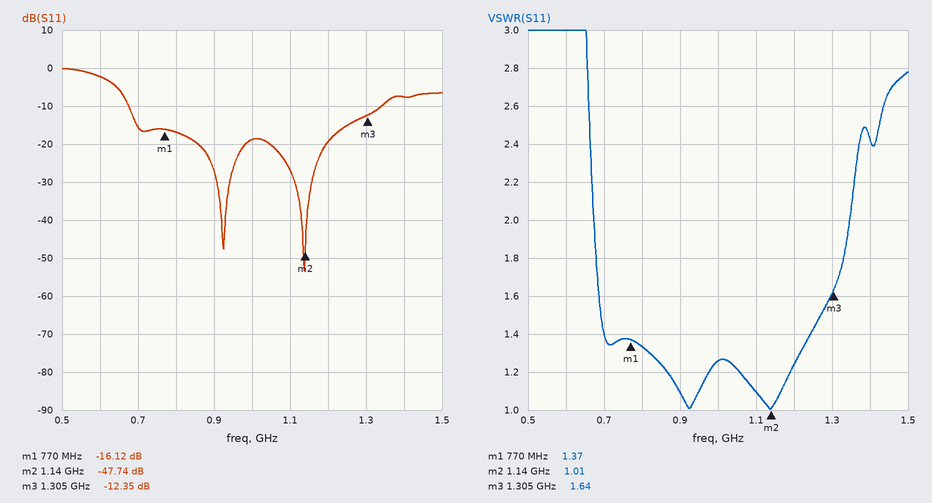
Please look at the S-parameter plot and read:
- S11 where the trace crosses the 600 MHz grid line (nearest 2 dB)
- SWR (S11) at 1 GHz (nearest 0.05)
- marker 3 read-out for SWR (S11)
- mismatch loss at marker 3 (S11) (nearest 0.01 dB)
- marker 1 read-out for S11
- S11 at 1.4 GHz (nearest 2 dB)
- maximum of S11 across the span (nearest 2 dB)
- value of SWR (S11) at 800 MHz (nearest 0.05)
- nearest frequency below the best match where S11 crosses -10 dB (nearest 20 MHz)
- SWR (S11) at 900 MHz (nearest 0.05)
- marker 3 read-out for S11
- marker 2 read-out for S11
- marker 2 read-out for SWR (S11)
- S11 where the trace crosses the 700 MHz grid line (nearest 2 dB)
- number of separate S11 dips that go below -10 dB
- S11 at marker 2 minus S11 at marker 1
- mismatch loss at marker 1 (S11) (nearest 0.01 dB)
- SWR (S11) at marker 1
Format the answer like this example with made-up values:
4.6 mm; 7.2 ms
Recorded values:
-2 dB; 1.25; 1.64; 0.26 dB; -16.12 dB; -8 dB; 0 dB; 1.35; 680 MHz; 1.10; -12.35 dB; -47.74 dB; 1.01; -16 dB; 2; -31.62 dB; 0.11 dB; 1.37
